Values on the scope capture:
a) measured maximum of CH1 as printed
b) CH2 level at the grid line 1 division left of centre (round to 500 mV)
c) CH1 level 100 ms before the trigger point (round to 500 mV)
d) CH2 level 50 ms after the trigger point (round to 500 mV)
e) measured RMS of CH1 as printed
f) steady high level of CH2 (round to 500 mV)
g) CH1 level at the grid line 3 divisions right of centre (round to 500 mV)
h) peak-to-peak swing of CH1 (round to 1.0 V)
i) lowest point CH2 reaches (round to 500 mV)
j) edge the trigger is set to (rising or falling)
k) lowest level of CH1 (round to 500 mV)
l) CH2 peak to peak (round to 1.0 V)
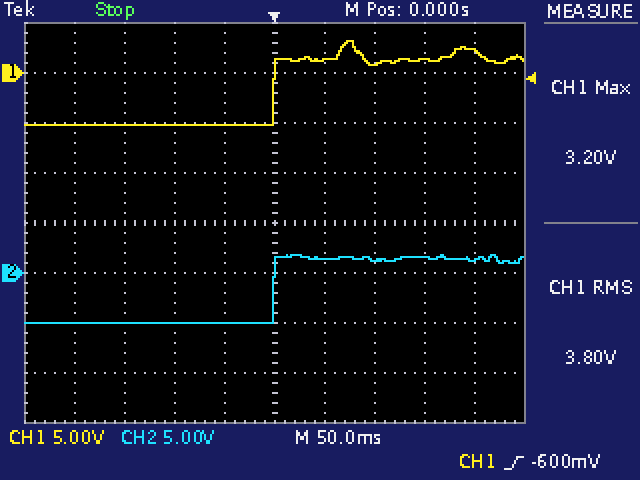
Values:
3.20 V
-5.0 V
-5.0 V
1.5 V
3.80 V
1.5 V
1.5 V
8.0 V
-5.0 V
rising
-5.0 V
7.0 V
